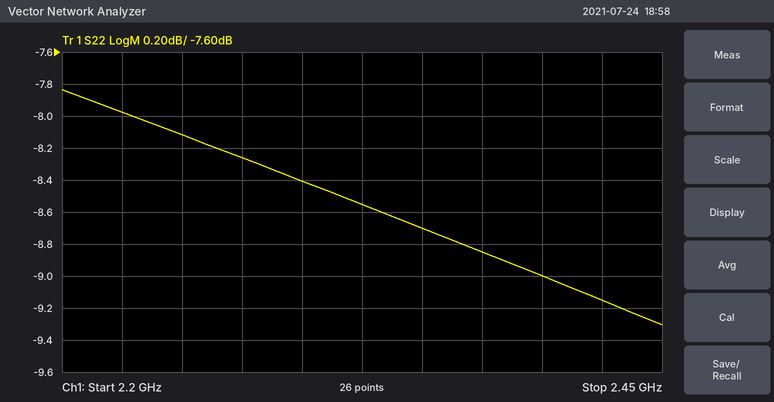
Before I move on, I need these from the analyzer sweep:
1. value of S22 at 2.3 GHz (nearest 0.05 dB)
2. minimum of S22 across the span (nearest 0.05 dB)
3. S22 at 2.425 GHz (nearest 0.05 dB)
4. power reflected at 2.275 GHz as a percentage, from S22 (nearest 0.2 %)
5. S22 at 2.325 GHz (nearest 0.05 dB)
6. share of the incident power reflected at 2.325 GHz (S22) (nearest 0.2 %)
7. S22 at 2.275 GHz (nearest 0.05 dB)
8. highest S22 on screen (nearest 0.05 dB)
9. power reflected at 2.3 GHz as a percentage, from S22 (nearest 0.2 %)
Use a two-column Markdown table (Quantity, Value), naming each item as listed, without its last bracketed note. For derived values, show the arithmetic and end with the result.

| Quantity | Value |
|---|---|
| value of S22 at 2.3 GHz | -8.40 dB |
| minimum of S22 across the span | -9.30 dB |
| S22 at 2.425 GHz | -9.15 dB |
| power reflected at 2.275 GHz as a percentage, from S22 | 10^(-8.25/10) ≈ 15.0 % |
| S22 at 2.325 GHz | -8.55 dB |
| share of the incident power reflected at 2.325 GHz (S22) | 10^(-8.55/10) ≈ 14.0 % |
| S22 at 2.275 GHz | -8.25 dB |
| highest S22 on screen | -7.85 dB |
| power reflected at 2.3 GHz as a percentage, from S22 | 10^(-8.4/10) ≈ 14.5 %, so 14.4 % to the nearest 0.2 % |
